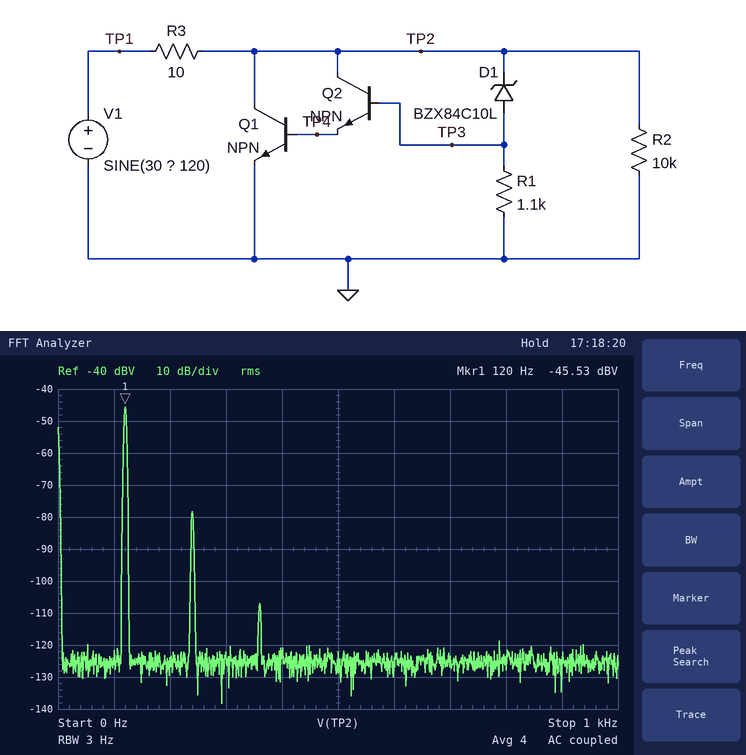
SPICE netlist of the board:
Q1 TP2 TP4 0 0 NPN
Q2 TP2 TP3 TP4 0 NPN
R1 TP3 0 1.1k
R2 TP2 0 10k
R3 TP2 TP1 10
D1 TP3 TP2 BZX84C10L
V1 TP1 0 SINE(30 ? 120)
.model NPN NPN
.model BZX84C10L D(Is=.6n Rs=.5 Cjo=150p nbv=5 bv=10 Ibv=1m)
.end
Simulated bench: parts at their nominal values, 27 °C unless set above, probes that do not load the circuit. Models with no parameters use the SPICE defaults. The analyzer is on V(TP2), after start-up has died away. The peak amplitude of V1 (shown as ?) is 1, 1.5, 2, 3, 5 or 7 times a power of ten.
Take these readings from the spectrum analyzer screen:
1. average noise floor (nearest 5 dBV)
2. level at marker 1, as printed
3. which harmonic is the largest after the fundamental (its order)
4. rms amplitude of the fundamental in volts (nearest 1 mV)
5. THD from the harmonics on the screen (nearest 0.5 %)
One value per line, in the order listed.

-125 dBV
-45.53 dBV
2
5 mV
2.5 %
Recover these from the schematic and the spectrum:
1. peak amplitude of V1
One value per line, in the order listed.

2 V
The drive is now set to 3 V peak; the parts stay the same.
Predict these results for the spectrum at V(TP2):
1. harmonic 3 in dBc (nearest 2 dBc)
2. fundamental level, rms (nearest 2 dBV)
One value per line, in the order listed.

-54 dBc
-42 dBV
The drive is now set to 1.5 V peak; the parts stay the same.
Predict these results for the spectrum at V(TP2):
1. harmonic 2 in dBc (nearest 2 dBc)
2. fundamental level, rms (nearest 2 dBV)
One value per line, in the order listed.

-36 dBc
-48 dBV
